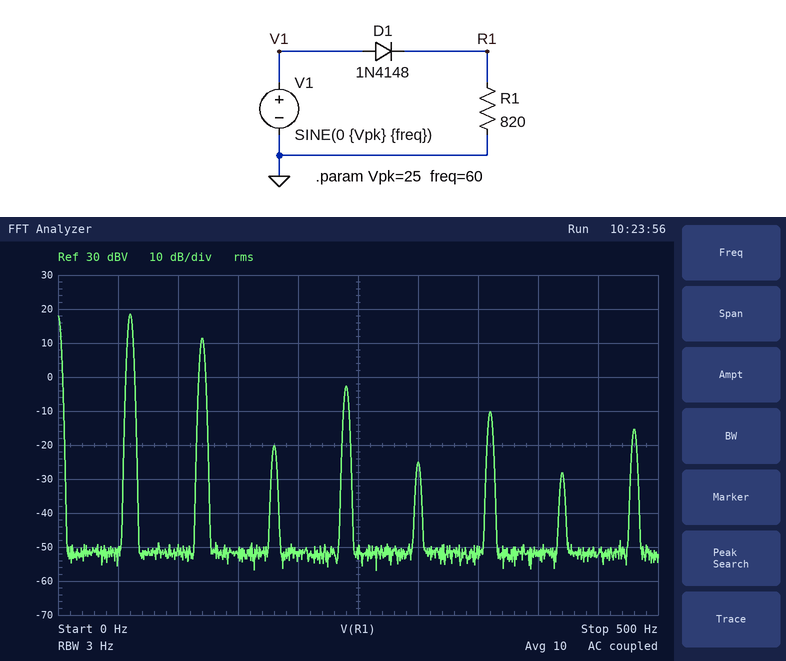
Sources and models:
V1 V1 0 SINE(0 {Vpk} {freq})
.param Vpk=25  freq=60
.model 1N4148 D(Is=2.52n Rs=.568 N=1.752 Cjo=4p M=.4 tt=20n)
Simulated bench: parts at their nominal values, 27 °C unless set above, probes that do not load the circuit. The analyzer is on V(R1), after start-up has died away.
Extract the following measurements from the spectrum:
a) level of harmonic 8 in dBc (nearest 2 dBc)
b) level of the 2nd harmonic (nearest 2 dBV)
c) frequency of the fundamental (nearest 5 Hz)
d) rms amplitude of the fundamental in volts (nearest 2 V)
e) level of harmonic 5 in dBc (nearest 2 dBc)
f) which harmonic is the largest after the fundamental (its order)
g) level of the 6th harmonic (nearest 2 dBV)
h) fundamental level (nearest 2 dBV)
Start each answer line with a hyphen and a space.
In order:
- -34 dBc
- 12 dBV
- 60 Hz
- 8 V
- -44 dBc
- 2
- -10 dBV
- 18 dBV
